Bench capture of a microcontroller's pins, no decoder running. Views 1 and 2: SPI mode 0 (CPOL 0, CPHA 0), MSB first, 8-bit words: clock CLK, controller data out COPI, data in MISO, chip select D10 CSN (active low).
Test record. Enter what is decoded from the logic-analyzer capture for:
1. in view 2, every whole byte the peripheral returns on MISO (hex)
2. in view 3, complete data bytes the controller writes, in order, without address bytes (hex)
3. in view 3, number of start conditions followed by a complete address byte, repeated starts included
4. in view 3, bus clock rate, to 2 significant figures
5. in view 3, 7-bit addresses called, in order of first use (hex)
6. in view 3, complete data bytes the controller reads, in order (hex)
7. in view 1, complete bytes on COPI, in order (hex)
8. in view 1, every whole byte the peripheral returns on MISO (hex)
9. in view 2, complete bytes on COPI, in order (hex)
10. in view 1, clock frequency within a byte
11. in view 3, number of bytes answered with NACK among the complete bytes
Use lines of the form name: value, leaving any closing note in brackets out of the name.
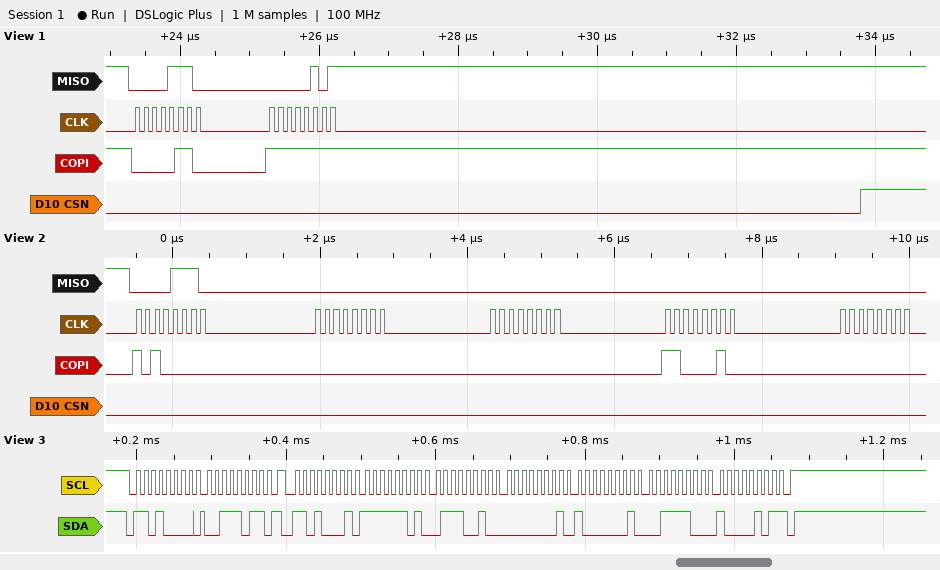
in view 2, every whole byte the peripheral returns on MISO: 0E 00 00 00 00
in view 3, complete data bytes the controller writes, in order, without address bytes: 3B
in view 3, number of start conditions followed by a complete address byte, repeated starts included: 2
in view 3, bus clock rate, to 2 significant figures: 100 kHz
in view 3, 7-bit addresses called, in order of first use: 0x68
in view 3, complete data bytes the controller reads, in order: FD 72 01 81 3C 85
in view 1, complete bytes on COPI, in order: 06 FF
in view 1, every whole byte the peripheral returns on MISO: 0E 05
in view 2, complete bytes on COPI, in order: A0 00 00 C2 00
in view 1, clock frequency within a byte: 8 MHz
in view 3, number of bytes answered with NACK among the complete bytes: 1
